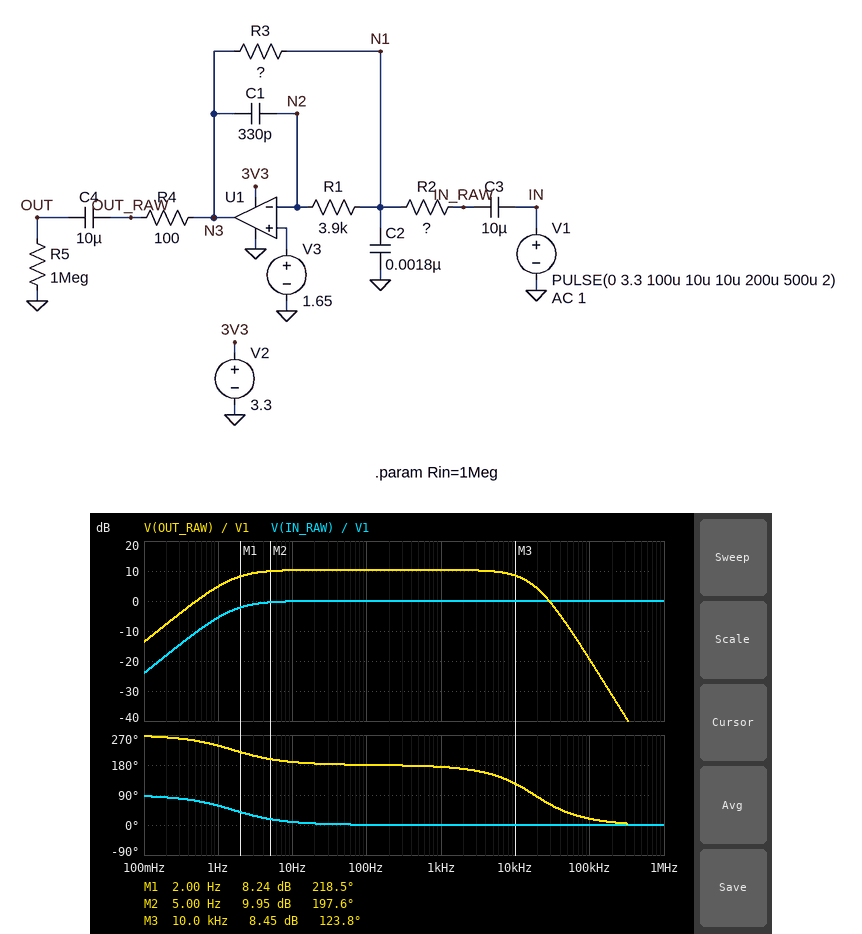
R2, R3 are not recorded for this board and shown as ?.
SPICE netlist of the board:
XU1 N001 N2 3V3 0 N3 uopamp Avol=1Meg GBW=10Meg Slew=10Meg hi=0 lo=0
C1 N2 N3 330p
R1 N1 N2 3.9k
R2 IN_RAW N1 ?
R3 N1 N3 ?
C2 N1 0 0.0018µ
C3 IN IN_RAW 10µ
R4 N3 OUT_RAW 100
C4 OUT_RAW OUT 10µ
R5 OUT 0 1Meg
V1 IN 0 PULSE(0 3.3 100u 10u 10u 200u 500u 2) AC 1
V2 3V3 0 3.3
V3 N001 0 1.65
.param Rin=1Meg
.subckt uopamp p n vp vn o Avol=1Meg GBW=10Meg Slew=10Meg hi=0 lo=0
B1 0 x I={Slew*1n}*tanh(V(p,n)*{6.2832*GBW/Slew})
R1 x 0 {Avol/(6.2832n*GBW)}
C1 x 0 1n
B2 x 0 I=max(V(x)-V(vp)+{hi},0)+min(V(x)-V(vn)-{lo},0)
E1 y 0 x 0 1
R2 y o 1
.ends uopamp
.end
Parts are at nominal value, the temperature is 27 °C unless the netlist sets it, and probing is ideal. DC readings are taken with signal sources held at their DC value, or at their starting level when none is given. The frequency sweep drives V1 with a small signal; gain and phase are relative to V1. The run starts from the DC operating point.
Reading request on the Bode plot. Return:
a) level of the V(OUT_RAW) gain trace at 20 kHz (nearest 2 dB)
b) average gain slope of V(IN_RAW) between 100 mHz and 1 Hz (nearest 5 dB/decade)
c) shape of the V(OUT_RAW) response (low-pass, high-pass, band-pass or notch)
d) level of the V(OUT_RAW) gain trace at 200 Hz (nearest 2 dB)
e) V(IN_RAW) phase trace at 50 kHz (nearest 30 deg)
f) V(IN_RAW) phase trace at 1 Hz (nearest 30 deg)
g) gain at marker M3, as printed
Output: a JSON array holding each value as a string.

["4 dB", "20 dB/decade", "band-pass", "10 dB", "0 deg", "60 deg", "8.45 dB"]
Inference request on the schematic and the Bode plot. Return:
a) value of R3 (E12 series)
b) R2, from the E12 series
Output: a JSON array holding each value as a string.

["33 kΩ", "10 kΩ"]
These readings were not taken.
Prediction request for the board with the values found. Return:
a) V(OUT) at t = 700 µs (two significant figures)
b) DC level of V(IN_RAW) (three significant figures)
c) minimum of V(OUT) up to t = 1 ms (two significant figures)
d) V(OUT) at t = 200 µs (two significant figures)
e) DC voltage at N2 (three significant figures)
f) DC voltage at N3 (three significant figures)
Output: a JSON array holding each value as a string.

["-1.7 V", "1.65 V", "-1.7 V", "-1.7 V", "1.65 V", "1.65 V"]
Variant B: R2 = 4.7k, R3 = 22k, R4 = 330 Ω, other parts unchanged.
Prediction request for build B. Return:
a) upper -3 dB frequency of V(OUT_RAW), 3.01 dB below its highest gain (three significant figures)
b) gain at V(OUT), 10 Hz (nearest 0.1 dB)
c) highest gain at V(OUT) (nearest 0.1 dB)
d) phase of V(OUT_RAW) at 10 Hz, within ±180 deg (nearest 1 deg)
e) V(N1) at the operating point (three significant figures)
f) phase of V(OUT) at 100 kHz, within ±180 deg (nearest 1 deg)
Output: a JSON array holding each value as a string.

["13.9 kHz", "12.9 dB", "13.4 dB", "-161 deg", "1.65 V", "25 deg"]
